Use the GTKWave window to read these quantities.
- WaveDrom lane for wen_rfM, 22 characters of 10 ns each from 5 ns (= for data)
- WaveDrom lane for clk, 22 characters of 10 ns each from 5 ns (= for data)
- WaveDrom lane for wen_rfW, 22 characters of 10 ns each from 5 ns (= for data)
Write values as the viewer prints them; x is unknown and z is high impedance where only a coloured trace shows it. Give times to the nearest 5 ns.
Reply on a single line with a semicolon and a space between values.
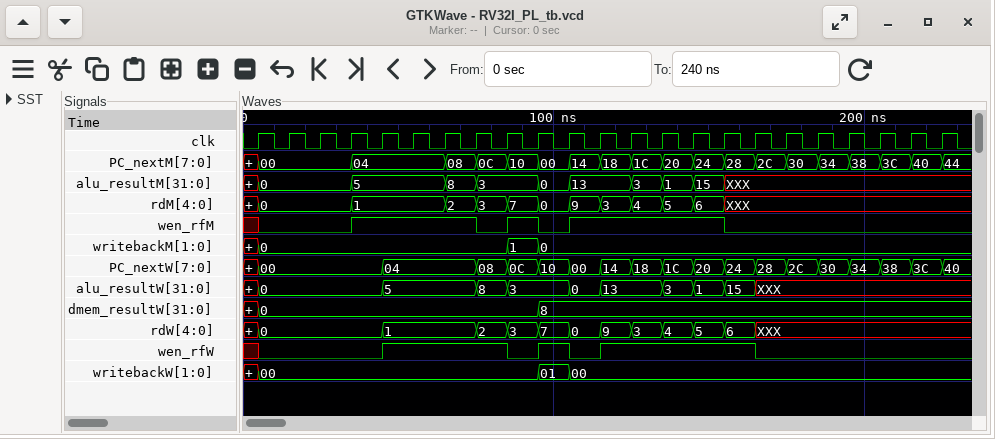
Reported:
{name: 'wen_rfM', wave: '0..1...0101....0......'}; {name: 'clk', wave: 'p.....................'}; {name: 'wen_rfW', wave: '0...1...0101....0.....'}
